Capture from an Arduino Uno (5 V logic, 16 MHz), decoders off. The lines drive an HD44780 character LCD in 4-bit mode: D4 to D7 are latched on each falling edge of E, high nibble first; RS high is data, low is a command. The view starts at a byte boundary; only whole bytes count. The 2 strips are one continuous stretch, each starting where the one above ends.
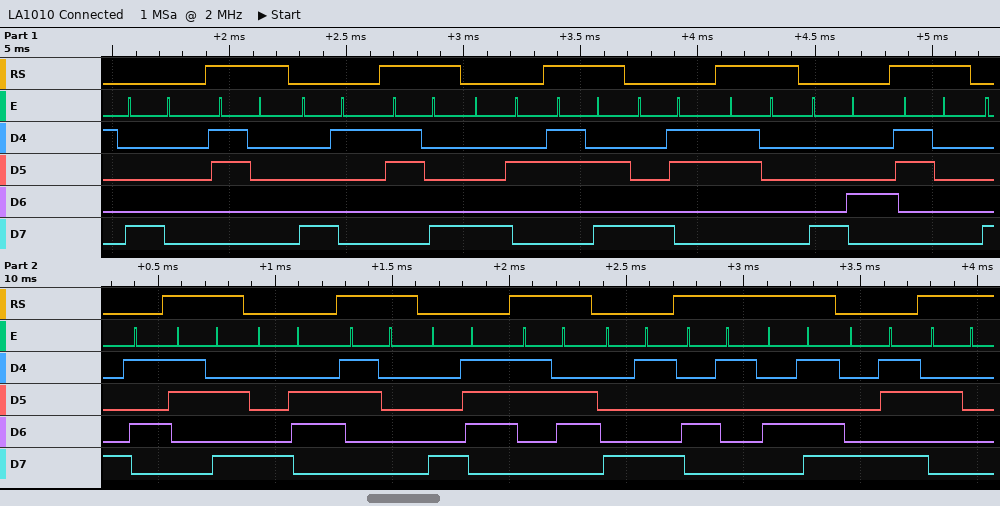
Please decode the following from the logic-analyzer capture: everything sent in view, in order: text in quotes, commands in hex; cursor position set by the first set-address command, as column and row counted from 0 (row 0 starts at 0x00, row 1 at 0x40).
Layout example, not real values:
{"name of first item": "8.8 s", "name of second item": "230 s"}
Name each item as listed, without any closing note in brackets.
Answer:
{"everything sent in view, in order: text in quotes, commands in hex": "0x80 \"0\" 0x81 \"8\" 0x82 \":\" 0x83 \"0\" 0x84 \"0\" 0x85 \":\" 0x86 \"0\" 0x87 \"6\" 0x89 \"AM\" 0x8B \" \"", "cursor position set by the first set-address command, as column and row counted from 0": "column 0, row 0"}
